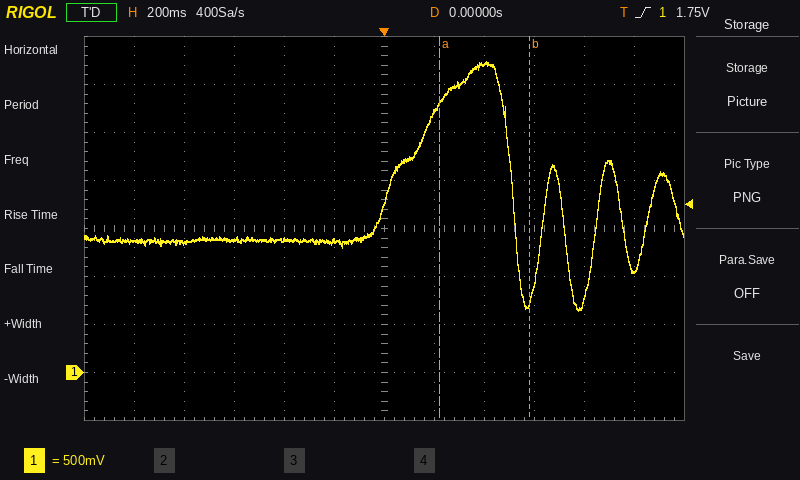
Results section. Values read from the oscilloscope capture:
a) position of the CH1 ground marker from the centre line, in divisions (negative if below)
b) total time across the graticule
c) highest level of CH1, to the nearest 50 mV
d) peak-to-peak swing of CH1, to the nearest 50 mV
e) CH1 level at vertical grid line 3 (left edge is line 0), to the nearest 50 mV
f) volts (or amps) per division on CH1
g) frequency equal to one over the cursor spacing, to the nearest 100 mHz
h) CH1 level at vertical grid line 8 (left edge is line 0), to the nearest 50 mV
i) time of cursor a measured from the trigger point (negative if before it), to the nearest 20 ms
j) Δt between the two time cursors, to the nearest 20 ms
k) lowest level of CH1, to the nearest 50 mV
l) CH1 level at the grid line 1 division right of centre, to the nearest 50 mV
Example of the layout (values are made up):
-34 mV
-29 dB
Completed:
-3.0 div
2.4 s
3.25 V
2.60 V
1.40 V
500 mV
2.8 Hz
3.20 V
+220 ms
360 ms
650 mV
2.70 V
